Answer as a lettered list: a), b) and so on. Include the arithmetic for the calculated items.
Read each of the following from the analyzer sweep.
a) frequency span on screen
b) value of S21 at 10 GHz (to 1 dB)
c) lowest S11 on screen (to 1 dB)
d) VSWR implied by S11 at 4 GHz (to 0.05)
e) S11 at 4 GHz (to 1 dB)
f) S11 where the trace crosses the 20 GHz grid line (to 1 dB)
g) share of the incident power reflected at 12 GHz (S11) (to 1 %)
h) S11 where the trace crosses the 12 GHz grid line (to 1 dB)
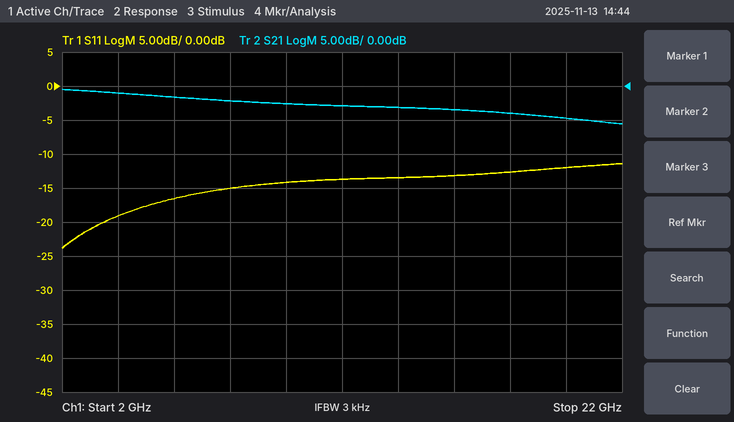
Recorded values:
a) 20 GHz
b) -3 dB
c) -24 dB
d) |Γ| = 10^(-19/20) = 0.1122; VSWR = (1 + 0.1122)/(1 − 0.1122) ≈ 1.25
e) -19 dB
f) -12 dB
g) 10^(-14/10) ≈ 4 %
h) -14 dB
